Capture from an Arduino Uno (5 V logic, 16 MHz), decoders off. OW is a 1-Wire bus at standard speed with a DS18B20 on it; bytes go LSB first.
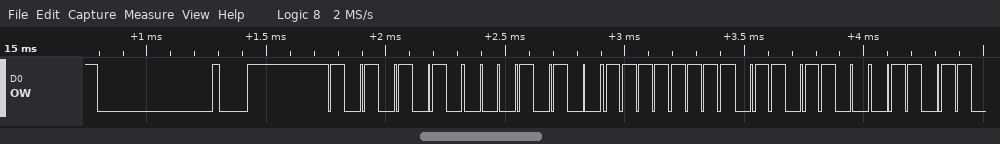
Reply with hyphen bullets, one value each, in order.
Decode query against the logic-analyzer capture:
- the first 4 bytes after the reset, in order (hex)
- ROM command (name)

- 55 28 FF 36
- Match ROM
